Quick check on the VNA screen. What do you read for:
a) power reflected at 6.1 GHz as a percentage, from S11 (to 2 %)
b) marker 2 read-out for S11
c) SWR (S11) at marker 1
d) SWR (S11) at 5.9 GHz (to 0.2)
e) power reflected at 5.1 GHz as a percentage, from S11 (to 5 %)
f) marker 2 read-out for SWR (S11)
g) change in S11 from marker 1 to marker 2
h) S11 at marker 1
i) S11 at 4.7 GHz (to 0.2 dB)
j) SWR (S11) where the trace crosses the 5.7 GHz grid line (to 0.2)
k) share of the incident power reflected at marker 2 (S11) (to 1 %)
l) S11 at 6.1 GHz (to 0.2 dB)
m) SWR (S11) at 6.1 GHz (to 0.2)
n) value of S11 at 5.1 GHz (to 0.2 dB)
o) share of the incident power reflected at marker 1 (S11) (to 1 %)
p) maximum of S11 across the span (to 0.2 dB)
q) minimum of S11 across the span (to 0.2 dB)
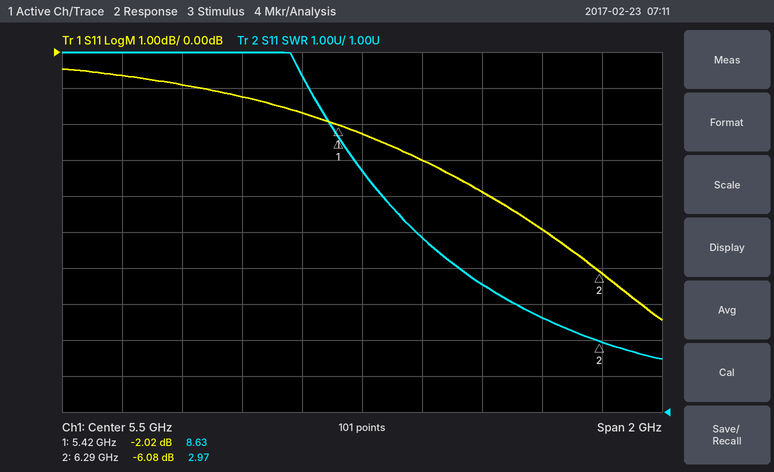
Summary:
32 %
-6.08 dB
8.63
4.6
75 %
2.97
-4.06 dB
-2.02 dB
-0.6 dB
5.8
25 %
-5.0 dB
3.6
-1.2 dB
63 %
-0.4 dB
-7.4 dB
